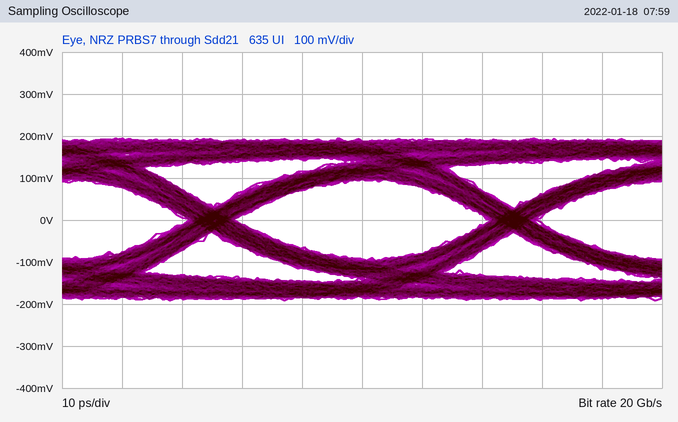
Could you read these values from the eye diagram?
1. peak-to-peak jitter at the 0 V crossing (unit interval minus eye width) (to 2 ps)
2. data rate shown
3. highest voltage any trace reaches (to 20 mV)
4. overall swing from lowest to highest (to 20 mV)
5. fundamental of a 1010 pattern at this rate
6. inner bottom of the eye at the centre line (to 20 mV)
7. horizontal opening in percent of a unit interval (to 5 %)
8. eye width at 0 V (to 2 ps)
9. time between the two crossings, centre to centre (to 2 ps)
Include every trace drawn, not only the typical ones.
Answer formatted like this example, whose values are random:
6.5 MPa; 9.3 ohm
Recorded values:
8 ps; 20 Gb/s; 200 mV; 380 mV; 10 GHz; -100 mV; 85 %; 42 ps; 50 ps
